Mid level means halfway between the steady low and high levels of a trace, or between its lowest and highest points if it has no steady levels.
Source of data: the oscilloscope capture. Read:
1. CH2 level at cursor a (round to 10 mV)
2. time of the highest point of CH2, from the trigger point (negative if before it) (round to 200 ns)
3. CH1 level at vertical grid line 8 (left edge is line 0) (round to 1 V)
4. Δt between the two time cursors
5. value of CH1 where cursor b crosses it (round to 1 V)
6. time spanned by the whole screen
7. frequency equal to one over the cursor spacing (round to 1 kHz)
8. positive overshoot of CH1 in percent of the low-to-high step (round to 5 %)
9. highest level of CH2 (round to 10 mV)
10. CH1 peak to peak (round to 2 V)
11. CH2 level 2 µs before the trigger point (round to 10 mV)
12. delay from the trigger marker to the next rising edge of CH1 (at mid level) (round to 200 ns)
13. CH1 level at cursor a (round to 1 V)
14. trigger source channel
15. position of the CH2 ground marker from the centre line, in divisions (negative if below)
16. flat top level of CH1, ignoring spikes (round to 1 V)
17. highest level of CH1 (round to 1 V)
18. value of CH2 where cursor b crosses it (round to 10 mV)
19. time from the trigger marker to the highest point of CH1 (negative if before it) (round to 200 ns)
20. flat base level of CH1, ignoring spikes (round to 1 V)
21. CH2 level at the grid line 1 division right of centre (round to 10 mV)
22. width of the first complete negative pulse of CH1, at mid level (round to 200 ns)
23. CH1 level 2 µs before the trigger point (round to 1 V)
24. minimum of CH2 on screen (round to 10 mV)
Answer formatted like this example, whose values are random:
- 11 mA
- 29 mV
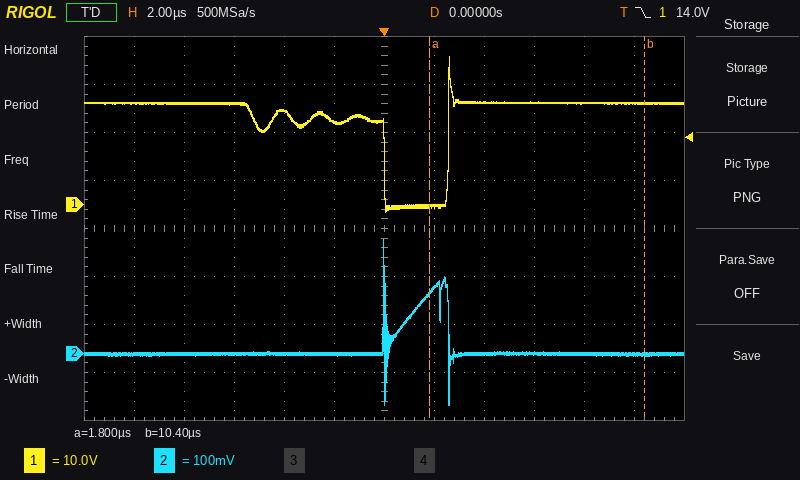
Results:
- 130 mV
- 0.0 µs
- 21 V
- 8.6 µs
- 21 V
- 24 µs
- 116 kHz
- 45 %
- 240 mV
- 32 V
- 0 mV
- 2.6 µs
- 0 V
- CH1
- -2.6 div
- 21 V
- 31 V
- 0 mV
- +2.6 µs
- 0 V
- 140 mV
- 2.6 µs
- 17 V
- -110 mV
